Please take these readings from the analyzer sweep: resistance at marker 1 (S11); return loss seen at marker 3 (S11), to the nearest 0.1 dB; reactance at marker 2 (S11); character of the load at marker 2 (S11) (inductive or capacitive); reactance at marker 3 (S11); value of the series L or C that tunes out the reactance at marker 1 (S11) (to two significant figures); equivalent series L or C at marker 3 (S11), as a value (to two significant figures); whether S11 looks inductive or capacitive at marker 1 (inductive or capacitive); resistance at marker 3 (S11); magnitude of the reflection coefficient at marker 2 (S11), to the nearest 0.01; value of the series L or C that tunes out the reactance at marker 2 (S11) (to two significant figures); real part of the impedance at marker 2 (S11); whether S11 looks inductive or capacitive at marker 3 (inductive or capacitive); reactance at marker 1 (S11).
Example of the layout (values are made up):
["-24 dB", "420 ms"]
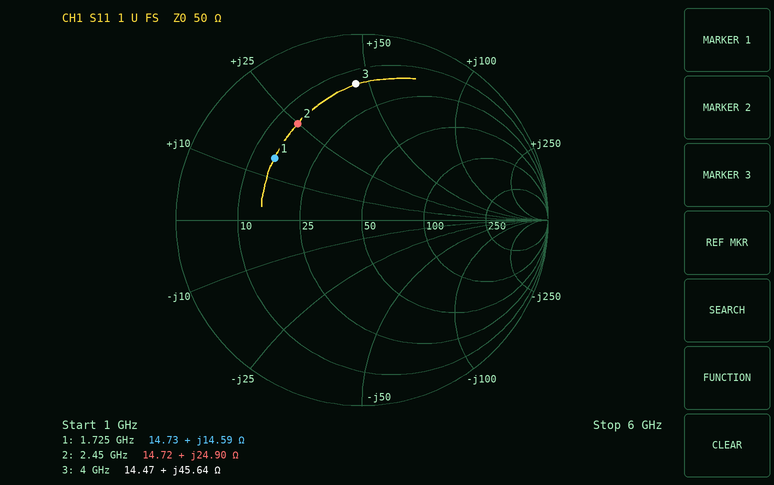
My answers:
["14.73 Ω", "2.7 dB", "+24.90 Ω", "inductive", "+45.64 Ω", "6.3 pF", "1.8 nH", "inductive", "14.47 Ω", "0.62", "2.6 pF", "14.72 Ω", "inductive", "+14.59 Ω"]
